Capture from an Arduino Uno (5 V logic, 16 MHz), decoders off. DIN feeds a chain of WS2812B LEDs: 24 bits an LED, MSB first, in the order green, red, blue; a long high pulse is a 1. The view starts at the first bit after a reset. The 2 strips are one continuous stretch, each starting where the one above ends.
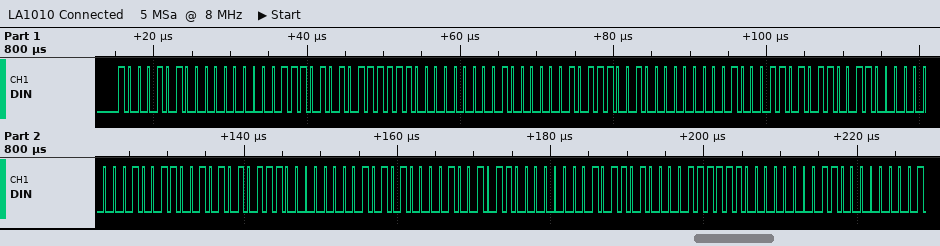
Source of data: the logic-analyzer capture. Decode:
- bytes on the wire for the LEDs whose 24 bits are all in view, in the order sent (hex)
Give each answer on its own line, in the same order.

8A 00 75 7E 00 81 72 00 8D 66 00 99 57 00 A8 4B 00 B4 3F 00 C0
